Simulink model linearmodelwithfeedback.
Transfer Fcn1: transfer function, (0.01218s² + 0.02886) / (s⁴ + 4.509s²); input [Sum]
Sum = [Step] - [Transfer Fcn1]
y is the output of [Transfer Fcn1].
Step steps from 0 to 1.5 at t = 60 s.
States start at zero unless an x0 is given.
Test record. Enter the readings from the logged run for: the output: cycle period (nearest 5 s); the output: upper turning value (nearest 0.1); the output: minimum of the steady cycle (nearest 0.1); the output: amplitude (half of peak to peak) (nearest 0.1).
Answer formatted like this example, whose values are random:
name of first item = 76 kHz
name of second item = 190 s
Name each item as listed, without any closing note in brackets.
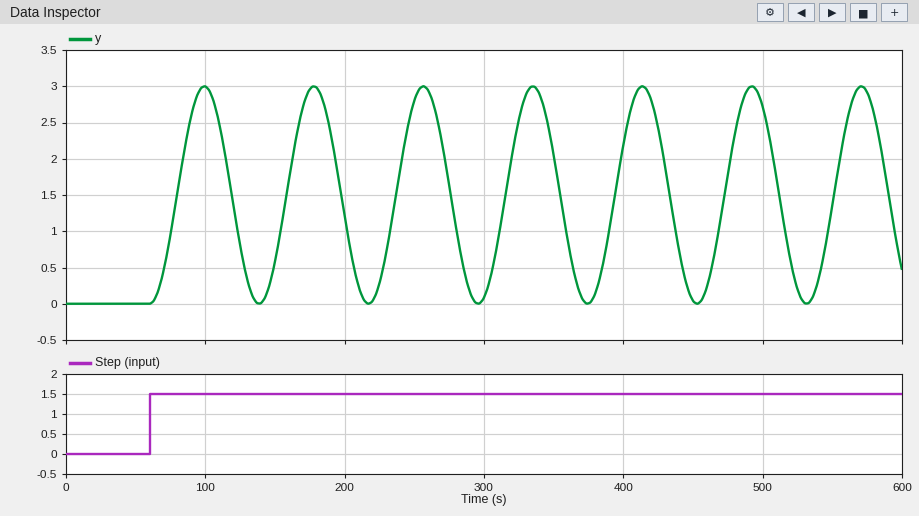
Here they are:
the output: cycle period = 80 s
the output: upper turning value = 3.0
the output: minimum of the steady cycle = 0.0
the output: amplitude (half of peak to peak) = 1.5
